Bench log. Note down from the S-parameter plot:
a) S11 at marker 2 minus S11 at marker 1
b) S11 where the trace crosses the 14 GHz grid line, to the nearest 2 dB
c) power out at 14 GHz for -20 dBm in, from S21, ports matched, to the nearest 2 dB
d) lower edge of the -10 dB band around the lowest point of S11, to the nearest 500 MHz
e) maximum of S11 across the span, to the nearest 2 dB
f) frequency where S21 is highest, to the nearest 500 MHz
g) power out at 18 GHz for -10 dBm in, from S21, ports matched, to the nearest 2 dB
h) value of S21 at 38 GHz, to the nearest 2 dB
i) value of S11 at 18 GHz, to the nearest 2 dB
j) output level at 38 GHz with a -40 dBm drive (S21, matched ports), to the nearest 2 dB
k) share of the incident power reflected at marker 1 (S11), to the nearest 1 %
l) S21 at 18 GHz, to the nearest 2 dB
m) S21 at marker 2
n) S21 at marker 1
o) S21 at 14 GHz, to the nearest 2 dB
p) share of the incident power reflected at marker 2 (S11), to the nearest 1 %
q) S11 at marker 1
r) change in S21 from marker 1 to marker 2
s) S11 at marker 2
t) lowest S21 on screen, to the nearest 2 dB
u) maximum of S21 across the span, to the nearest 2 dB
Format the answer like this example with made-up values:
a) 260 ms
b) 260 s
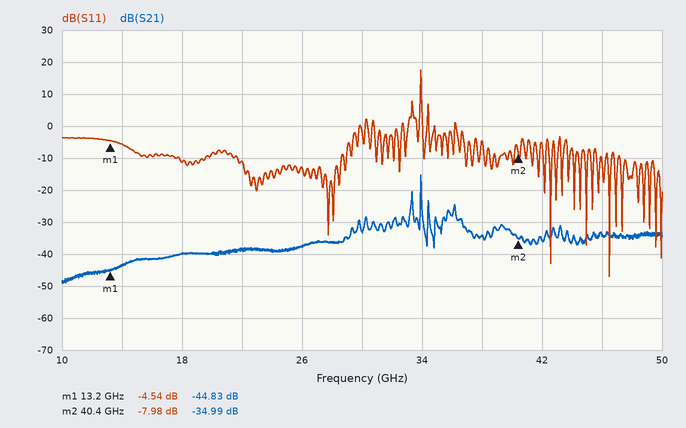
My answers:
a) -3.44 dB
b) -6 dB
c) -64 dBm
d) 46.5 GHz
e) 18 dB
f) 34.0 GHz
g) -50 dBm
h) -34 dB
i) -12 dB
j) -74 dBm
k) 35 %
l) -40 dB
m) -34.99 dB
n) -44.83 dB
o) -44 dB
p) 16 %
q) -4.54 dB
r) 9.84 dB
s) -7.98 dB
t) -50 dB
u) -16 dB
